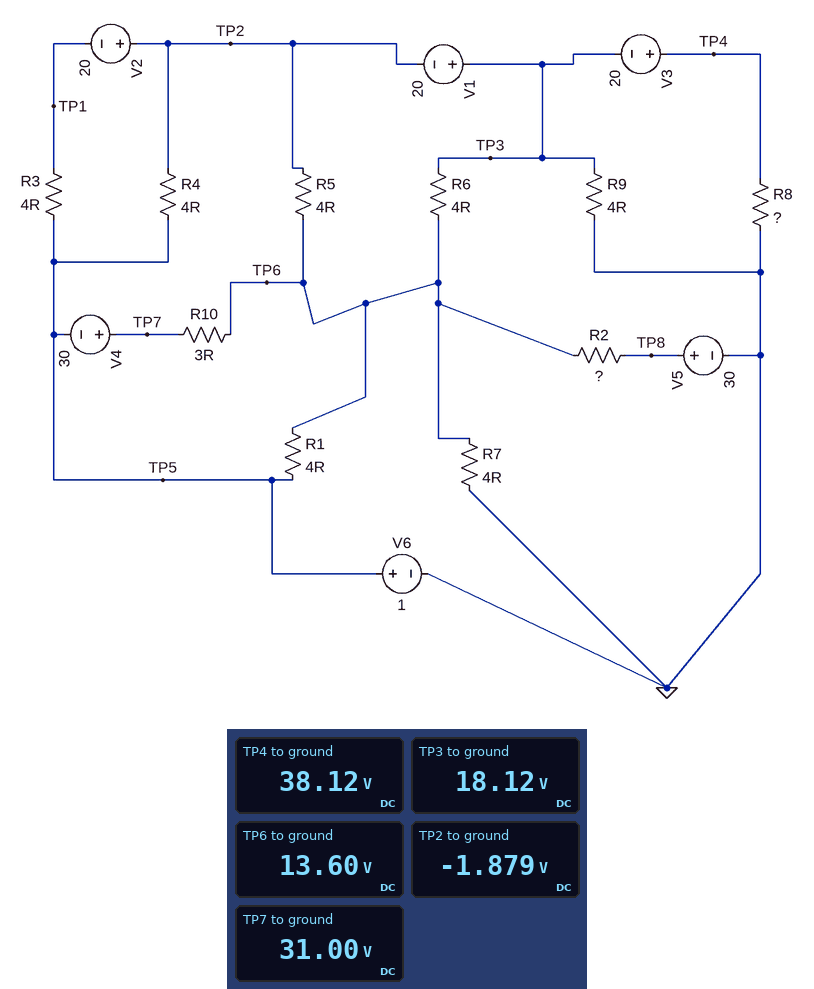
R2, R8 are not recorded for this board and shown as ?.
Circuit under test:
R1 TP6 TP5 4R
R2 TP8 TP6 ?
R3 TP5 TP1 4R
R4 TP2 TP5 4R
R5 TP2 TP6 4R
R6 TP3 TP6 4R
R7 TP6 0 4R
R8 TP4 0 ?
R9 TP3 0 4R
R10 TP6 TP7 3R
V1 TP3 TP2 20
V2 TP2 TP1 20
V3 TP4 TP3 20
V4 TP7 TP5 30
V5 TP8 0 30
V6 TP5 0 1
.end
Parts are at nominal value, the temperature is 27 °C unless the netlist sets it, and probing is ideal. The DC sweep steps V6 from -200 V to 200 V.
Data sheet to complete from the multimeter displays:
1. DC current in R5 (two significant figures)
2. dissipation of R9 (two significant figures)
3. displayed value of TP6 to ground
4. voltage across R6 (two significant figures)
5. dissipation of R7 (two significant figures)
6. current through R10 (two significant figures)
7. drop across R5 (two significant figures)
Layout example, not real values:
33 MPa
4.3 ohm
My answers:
3.9 A
82 W
13.60 V
4.5 V
46 W
5.8 A
15 V
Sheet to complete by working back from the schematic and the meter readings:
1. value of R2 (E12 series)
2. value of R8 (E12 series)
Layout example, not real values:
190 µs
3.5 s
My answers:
4.7 Ω
8.2 Ω
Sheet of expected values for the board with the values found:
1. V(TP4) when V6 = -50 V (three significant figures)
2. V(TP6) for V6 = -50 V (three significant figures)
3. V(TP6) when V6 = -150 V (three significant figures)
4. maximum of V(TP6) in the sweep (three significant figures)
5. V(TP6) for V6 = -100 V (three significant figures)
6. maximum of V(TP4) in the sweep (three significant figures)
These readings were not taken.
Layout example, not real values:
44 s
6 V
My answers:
9.10 V
-15.0 V
-71.2 V
125 V
-43.1 V
151 V
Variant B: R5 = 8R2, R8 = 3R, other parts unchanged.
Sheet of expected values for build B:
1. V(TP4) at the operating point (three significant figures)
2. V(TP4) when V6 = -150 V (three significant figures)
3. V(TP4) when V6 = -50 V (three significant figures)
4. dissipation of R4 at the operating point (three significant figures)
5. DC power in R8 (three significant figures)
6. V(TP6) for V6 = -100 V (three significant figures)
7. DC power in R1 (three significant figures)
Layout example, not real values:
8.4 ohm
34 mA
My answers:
31.1 V
-41.5 V
6.58 V
24.5 W
323 W
-41.1 V
37.0 W
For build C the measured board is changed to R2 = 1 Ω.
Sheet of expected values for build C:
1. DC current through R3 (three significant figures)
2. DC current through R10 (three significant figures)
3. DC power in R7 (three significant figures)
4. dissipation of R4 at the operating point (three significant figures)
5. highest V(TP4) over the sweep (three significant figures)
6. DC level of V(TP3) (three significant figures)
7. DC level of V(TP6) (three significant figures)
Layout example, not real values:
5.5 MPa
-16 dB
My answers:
5.17 A
3.80 A
96.1 W
120 mW
139 V
20.3 V
19.6 V
